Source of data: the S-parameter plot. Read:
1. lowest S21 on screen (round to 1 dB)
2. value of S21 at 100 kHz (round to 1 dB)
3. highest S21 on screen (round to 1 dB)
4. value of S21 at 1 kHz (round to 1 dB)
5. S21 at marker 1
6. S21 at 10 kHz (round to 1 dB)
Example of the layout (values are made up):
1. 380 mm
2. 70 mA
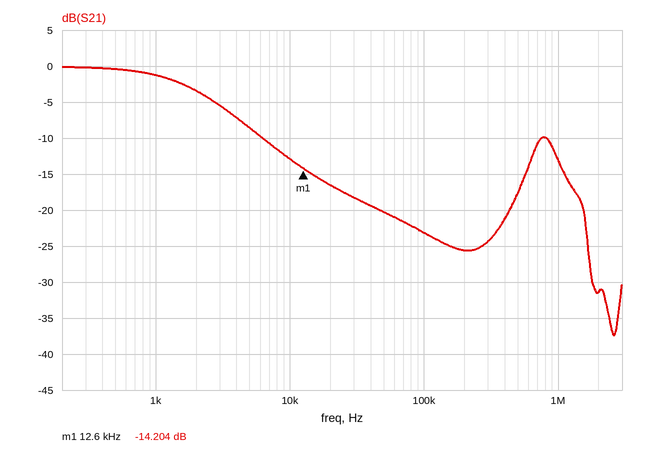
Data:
1. -37 dB
2. -23 dB
3. 0 dB
4. -1 dB
5. -14.204 dB
6. -13 dB
